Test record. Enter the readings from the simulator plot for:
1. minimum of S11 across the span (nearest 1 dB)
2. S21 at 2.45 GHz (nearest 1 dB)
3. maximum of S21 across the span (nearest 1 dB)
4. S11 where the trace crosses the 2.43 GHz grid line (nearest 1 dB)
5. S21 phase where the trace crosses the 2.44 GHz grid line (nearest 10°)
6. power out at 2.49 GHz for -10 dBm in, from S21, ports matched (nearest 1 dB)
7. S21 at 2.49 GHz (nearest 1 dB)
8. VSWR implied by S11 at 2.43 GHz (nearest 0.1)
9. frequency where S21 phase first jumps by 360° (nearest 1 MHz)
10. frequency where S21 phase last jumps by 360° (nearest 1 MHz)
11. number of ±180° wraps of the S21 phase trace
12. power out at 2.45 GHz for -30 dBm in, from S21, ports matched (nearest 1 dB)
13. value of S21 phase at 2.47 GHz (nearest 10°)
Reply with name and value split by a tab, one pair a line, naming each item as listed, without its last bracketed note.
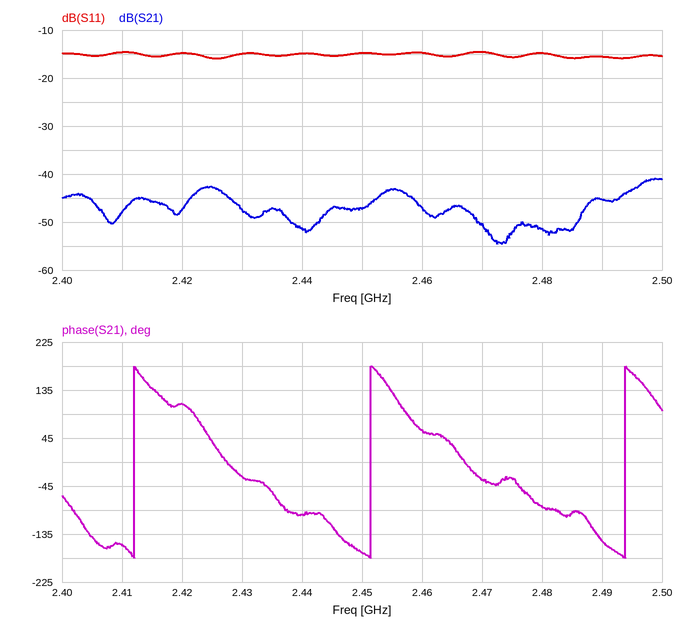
minimum of S11 across the span	-16 dB
S21 at 2.45 GHz	-47 dB
maximum of S21 across the span	-41 dB
S11 where the trace crosses the 2.43 GHz grid line	-15 dB
S21 phase where the trace crosses the 2.44 GHz grid line	-100°
power out at 2.49 GHz for -10 dBm in, from S21, ports matched	-55 dBm
S21 at 2.49 GHz	-45 dB
VSWR implied by S11 at 2.43 GHz	1.4
frequency where S21 phase first jumps by 360°	2.412 GHz
frequency where S21 phase last jumps by 360°	2.494 GHz
number of ±180° wraps of the S21 phase trace	3
power out at 2.45 GHz for -30 dBm in, from S21, ports matched	-77 dBm
value of S21 phase at 2.47 GHz	-30°
